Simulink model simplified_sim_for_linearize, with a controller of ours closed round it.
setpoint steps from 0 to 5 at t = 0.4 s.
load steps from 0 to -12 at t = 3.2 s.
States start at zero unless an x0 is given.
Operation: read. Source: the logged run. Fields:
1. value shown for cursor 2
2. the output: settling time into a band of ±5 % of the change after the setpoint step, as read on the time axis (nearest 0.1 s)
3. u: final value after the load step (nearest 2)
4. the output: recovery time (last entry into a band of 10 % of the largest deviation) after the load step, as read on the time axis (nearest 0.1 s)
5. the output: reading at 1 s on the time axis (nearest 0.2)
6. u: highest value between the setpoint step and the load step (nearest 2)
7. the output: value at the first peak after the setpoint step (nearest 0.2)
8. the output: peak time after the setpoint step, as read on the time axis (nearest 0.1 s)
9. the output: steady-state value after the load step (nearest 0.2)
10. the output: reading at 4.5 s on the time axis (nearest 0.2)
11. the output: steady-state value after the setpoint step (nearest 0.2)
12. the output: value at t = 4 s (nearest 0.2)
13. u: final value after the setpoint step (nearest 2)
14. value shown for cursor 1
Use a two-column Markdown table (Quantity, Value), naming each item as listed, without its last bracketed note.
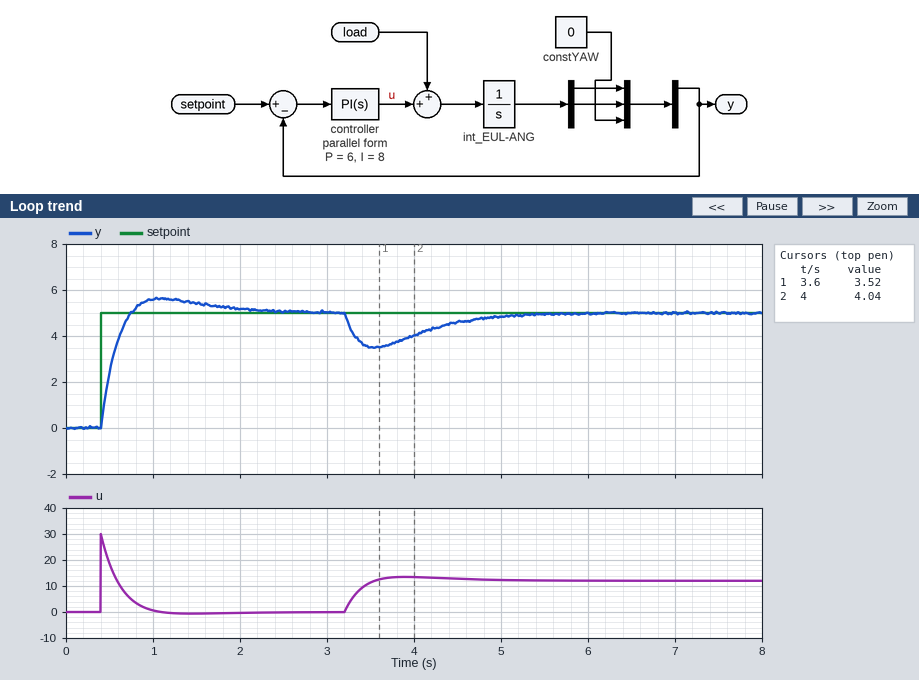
| Quantity | Value |
|---|---|
| value shown for cursor 2 | 4.04 |
| the output: settling time into a band of ±5 % of the change after the setpoint step, as read on the time axis | 1.8 s |
| u: final value after the load step | 12 |
| the output: recovery time (last entry into a band of 10 % of the largest deviation) after the load step, as read on the time axis | 5.0 s |
| the output: reading at 1 s on the time axis | 5.6 |
| u: highest value between the setpoint step and the load step | 30 |
| the output: value at the first peak after the setpoint step | 5.6 |
| the output: peak time after the setpoint step, as read on the time axis | 1.1 s |
| the output: steady-state value after the load step | 5.0 |
| the output: reading at 4.5 s on the time axis | 4.6 |
| the output: steady-state value after the setpoint step | 5.0 |
| the output: value at t = 4 s | 4.0 |
| u: final value after the setpoint step | 0 |
| value shown for cursor 1 | 3.52 |
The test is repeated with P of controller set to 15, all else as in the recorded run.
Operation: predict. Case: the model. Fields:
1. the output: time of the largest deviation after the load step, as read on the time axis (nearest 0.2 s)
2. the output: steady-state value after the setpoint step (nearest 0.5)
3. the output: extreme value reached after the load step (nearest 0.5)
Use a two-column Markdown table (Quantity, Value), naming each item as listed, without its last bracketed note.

| Quantity | Value |
|---|---|
| the output: time of the largest deviation after the load step, as read on the time axis | 3.4 s |
| the output: steady-state value after the setpoint step | 5.0 |
| the output: extreme value reached after the load step | 4.5 |
